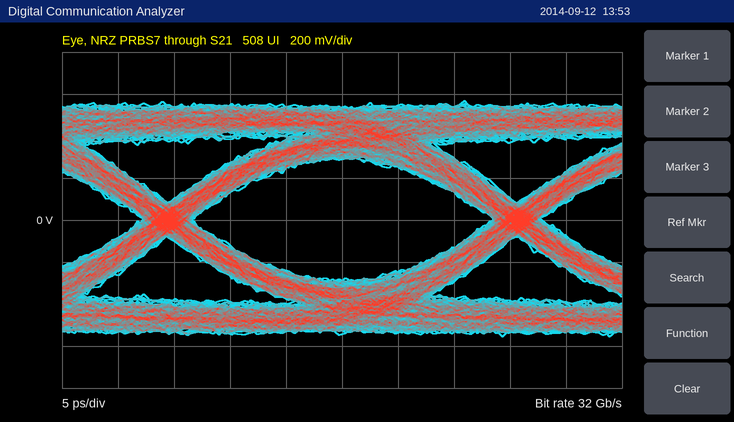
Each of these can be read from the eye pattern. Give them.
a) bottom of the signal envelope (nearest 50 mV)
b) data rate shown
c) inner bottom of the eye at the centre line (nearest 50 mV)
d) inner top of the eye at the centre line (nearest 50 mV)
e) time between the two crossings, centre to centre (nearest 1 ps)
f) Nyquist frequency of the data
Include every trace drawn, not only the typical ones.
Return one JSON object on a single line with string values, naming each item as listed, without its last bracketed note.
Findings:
{"bottom of the signal envelope": "-550 mV", "data rate shown": "32 Gb/s", "inner bottom of the eye at the centre line": "-300 mV", "inner top of the eye at the centre line": "300 mV", "time between the two crossings, centre to centre": "31 ps", "Nyquist frequency of the data": "16 GHz"}
